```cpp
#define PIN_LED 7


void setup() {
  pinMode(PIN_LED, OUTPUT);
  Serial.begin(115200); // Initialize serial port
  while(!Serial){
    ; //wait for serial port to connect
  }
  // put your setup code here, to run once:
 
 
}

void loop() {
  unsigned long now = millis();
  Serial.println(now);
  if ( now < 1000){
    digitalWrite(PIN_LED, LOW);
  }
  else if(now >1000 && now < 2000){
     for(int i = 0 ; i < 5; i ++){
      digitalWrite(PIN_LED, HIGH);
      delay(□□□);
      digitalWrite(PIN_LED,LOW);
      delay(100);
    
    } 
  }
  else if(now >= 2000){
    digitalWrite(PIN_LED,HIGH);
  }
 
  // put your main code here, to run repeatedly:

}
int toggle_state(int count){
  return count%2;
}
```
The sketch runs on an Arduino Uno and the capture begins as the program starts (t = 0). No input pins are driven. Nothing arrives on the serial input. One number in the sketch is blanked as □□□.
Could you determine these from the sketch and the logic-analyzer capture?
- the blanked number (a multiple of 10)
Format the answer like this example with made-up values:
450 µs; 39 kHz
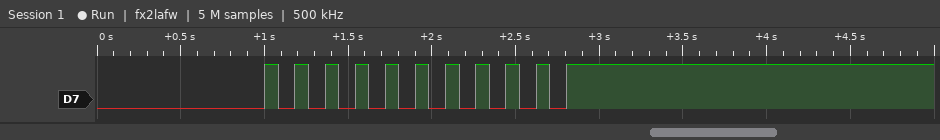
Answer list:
80
